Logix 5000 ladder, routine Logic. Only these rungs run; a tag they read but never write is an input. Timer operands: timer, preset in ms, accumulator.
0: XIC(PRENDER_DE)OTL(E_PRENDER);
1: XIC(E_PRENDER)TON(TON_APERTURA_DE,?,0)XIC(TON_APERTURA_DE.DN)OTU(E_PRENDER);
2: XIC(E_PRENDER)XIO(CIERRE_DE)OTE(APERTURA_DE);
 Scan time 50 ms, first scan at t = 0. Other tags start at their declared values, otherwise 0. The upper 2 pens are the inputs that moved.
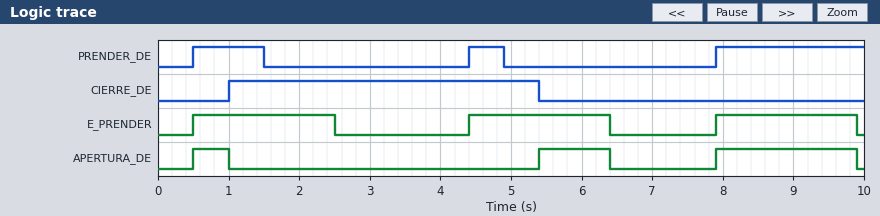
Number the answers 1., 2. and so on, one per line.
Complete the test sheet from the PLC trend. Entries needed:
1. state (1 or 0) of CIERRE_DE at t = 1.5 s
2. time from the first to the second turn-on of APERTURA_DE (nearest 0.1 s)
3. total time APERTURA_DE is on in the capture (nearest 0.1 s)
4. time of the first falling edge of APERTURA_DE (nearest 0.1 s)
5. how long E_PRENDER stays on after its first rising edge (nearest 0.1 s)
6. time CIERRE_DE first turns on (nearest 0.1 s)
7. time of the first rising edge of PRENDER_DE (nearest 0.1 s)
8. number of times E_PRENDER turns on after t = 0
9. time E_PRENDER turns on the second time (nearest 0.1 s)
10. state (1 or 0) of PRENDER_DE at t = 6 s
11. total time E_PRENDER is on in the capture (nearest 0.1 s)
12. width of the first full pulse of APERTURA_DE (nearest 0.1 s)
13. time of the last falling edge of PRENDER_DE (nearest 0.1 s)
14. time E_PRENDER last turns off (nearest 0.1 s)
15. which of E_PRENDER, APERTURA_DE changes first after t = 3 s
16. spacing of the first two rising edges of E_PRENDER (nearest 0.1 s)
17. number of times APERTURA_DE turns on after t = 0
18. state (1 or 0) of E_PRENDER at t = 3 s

1. 1
2. 4.9 s
3. 3.5 s
4. 1.0 s
5. 2.0 s
6. 1.0 s
7. 0.5 s
8. 3
9. 4.4 s
10. 0
11. 6.0 s
12. 0.5 s
13. 4.9 s
14. 9.9 s
15. E_PRENDER
16. 3.9 s
17. 3
18. 0
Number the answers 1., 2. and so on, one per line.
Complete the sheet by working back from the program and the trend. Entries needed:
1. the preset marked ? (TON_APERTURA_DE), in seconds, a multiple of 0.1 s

1. 2.0 s
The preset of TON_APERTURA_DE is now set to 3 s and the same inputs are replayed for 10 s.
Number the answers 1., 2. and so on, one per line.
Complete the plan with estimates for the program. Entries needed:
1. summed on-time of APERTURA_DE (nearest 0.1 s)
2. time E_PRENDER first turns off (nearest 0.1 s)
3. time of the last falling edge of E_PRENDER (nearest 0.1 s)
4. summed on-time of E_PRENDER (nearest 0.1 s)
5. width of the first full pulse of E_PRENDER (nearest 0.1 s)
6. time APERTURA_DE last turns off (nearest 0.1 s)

1. 4.6 s
2. 3.5 s
3. 7.4 s
4. 8.1 s
5. 3.0 s
6. 7.4 s
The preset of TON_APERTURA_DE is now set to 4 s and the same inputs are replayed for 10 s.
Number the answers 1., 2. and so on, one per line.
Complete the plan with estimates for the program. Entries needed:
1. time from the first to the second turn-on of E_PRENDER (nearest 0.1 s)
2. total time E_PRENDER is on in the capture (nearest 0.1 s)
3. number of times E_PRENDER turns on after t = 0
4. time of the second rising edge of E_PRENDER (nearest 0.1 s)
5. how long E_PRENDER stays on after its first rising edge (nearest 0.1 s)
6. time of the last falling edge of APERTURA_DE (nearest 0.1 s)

1. 7.4 s
2. 6.1 s
3. 2
4. 7.9 s
5. 4.0 s
6. 1.0 s
